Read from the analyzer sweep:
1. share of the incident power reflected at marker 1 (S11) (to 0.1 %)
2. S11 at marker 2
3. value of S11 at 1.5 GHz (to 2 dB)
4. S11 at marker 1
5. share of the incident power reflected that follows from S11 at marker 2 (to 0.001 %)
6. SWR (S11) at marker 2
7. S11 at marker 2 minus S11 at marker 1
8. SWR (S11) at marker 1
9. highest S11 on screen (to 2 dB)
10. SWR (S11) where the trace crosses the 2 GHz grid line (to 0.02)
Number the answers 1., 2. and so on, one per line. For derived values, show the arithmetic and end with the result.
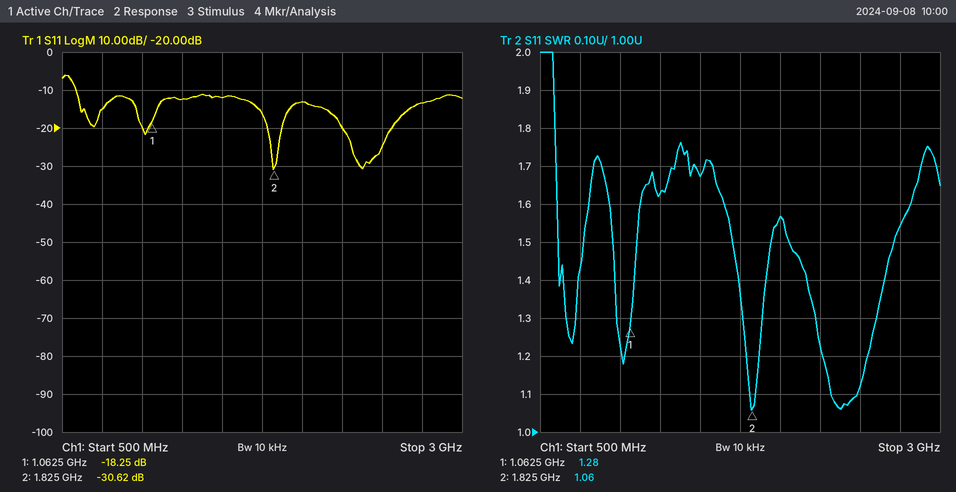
1. 10^(-18.25/10) ≈ 1.5 %
2. -30.62 dB
3. -12 dB
4. -18.25 dB
5. 10^(-30.62/10) ≈ 0.087 %
6. 1.06
7. -30.62 − (-18.25) = -12.37 dB
8. 1.28
9. -6 dB
10. 1.56
